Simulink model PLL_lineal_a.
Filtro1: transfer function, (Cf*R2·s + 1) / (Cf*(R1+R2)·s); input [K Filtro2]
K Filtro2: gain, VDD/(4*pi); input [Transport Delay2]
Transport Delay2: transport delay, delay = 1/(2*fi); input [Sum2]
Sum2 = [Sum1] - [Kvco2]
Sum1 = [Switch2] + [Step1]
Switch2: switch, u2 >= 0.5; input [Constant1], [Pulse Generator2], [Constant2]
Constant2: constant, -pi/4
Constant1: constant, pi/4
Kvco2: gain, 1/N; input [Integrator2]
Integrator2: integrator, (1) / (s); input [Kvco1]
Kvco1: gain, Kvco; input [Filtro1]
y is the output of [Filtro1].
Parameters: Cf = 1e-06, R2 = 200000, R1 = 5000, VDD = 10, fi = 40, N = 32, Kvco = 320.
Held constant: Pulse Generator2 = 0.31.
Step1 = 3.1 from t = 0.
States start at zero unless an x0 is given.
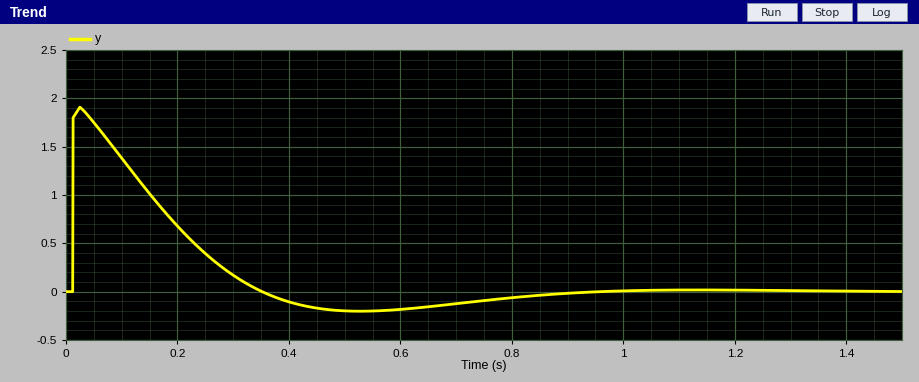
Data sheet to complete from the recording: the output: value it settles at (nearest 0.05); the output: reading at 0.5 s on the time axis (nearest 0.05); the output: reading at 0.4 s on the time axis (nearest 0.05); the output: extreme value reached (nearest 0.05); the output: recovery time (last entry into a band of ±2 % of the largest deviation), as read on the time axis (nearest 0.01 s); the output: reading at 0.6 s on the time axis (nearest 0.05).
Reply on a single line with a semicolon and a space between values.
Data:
0.00; -0.20; -0.10; 1.90; 0.85 s; -0.20
